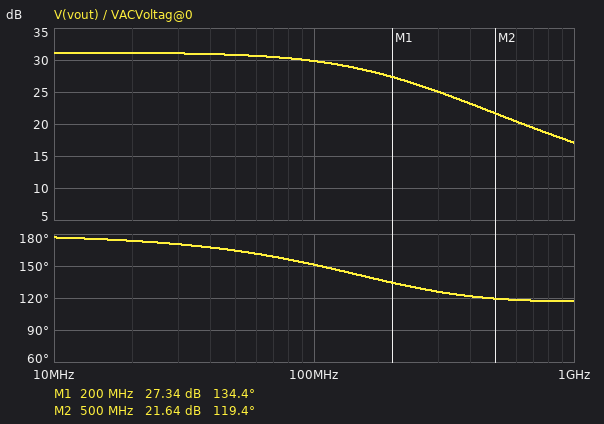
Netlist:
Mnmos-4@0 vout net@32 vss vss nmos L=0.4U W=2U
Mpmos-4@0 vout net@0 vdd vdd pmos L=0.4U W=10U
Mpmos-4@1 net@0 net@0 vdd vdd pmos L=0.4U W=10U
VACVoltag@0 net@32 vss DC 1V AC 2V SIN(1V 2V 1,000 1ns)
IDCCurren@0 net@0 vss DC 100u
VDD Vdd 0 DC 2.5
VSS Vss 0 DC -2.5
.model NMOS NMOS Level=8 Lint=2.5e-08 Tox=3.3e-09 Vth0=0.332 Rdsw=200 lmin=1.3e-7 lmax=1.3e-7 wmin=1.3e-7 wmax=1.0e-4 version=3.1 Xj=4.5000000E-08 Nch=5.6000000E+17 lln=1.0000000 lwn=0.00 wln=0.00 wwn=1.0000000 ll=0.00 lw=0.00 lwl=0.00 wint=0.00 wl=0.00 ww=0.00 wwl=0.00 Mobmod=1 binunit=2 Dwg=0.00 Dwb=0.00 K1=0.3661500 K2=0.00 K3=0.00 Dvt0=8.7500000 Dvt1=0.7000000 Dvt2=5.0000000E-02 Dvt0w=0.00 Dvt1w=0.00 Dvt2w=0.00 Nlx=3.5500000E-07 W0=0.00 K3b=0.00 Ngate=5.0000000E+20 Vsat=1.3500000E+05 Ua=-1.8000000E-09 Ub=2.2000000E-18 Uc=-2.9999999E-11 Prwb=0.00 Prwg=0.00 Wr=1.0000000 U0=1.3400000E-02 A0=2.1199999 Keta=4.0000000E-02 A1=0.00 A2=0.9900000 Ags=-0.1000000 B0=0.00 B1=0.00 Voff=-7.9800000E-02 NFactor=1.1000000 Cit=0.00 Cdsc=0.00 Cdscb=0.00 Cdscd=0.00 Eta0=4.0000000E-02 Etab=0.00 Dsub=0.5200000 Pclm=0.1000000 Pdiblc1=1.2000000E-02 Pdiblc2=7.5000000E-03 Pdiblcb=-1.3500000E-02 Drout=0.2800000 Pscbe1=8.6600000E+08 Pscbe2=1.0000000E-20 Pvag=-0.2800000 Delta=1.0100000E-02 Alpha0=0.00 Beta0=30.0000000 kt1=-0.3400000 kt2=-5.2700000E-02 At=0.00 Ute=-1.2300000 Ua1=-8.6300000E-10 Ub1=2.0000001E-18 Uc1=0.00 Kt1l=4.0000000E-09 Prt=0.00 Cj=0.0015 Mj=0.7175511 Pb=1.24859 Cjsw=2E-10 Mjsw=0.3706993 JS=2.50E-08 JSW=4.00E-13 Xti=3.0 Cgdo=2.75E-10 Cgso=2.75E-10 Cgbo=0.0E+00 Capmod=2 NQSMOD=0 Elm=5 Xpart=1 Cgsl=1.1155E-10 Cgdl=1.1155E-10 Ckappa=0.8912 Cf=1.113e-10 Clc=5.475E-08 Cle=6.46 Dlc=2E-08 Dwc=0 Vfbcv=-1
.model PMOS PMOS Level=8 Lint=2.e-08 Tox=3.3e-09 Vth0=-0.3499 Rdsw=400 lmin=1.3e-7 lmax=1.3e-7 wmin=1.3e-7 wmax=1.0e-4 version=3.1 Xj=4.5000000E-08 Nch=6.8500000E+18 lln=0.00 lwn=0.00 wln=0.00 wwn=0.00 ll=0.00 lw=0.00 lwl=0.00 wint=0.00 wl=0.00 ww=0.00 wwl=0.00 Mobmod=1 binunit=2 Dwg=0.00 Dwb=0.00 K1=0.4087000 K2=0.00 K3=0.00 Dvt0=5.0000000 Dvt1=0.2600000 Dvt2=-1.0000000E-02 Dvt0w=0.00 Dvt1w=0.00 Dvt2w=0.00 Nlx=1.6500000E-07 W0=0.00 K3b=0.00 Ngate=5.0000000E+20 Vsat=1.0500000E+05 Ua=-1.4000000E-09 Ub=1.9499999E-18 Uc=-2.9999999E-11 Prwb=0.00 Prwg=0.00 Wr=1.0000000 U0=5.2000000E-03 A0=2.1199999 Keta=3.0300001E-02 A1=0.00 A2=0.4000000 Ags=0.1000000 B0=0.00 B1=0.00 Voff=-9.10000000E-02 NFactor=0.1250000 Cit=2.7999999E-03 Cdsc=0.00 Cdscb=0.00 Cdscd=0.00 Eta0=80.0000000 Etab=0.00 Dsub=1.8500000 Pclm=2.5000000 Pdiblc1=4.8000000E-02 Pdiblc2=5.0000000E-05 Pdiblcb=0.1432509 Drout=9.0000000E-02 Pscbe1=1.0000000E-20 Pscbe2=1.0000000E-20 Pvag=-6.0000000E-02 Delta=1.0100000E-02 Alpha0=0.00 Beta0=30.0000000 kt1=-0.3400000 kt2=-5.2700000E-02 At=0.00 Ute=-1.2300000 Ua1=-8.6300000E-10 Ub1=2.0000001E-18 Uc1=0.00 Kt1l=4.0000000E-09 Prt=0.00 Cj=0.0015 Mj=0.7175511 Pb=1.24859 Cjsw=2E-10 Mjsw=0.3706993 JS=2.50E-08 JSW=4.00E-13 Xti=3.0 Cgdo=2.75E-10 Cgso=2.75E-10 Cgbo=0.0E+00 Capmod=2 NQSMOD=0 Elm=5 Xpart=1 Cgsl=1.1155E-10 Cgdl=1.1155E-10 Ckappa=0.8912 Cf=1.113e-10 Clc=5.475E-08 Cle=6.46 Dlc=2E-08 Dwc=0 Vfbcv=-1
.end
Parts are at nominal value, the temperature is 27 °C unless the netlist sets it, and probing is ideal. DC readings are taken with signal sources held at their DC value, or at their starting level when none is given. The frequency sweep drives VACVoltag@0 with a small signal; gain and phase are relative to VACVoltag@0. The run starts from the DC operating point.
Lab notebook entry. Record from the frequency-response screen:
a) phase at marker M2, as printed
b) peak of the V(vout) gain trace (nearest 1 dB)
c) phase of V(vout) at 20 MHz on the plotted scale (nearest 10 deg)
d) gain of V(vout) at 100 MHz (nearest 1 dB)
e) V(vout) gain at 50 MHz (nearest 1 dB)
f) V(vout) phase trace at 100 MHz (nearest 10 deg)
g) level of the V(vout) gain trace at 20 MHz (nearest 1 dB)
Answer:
119.4 deg
31 dB
170 deg
30 dB
31 dB
150 deg
31 dB
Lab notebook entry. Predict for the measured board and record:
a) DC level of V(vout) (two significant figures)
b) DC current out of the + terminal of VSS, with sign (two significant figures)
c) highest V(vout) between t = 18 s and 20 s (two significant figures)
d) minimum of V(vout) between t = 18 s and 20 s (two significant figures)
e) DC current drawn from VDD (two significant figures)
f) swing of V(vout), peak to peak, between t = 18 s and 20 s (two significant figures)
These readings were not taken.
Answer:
-1.7 V
-230 µA
2.5 V
-2.4 V
230 µA
4.9 V
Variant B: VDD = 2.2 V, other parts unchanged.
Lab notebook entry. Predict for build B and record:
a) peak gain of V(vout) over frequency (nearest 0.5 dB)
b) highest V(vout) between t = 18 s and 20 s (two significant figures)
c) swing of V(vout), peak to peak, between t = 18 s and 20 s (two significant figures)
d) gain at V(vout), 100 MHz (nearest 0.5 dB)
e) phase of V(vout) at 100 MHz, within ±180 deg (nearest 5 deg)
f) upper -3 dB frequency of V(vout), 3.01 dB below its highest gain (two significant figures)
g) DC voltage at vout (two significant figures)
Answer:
30.0 dB
2.2 V
4.6 V
29.0 dB
155 deg
190 MHz
-1.8 V
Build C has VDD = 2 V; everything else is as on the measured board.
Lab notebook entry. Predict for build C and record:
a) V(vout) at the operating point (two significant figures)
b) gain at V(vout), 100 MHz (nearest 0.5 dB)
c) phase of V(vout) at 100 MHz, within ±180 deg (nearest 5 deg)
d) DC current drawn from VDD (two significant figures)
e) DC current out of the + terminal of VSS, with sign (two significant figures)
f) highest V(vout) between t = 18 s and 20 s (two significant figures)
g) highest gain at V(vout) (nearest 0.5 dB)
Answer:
-1.9 V
27.5 dB
160 deg
220 µA
-220 µA
2.0 V
28.0 dB
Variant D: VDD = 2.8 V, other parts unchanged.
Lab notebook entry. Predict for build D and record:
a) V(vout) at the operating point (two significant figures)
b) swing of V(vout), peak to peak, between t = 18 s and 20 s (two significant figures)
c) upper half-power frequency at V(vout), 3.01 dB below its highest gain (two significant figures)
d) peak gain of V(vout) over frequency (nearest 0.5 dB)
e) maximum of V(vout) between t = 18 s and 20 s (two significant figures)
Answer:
-1.5 V
5.2 V
160 MHz
31.5 dB
2.8 V
